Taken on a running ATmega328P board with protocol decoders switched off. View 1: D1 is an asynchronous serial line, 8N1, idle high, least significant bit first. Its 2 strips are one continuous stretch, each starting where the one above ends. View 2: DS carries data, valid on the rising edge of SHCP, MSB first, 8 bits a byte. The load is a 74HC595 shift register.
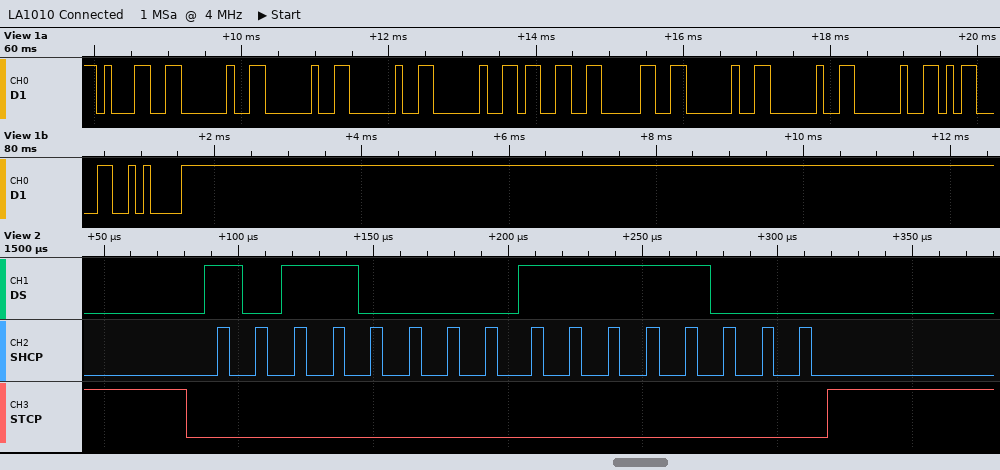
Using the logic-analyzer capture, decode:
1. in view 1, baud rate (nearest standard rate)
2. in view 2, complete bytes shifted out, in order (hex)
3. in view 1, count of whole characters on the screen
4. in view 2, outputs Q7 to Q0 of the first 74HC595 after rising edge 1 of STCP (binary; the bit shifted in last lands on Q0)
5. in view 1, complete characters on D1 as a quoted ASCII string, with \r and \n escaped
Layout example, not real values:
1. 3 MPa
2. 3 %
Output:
1. 9600 baud
2. 0xB0 0xF8
3. 12
4. 11111000
5. "1    30   \r\n"
